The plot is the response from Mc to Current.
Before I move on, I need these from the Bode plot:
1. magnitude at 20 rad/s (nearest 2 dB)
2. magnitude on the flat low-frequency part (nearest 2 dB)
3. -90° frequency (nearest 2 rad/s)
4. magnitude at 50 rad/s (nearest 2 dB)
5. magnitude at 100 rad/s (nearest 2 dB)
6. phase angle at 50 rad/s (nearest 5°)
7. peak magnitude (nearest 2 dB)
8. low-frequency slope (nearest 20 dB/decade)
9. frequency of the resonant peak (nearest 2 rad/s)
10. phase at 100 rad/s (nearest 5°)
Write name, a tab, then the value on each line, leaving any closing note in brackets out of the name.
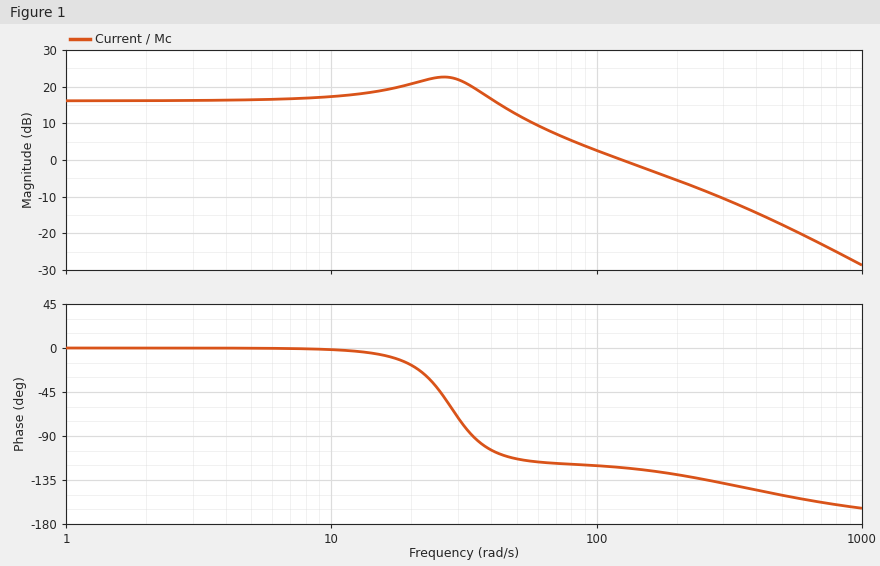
magnitude at 20 rad/s	20 dB
magnitude on the flat low-frequency part	16 dB
-90° frequency	34 rad/s
magnitude at 50 rad/s	12 dB
magnitude at 100 rad/s	2 dB
phase angle at 50 rad/s	-115°
peak magnitude	22 dB
low-frequency slope	0 dB/decade
frequency of the resonant peak	26 rad/s
phase at 100 rad/s	-120°
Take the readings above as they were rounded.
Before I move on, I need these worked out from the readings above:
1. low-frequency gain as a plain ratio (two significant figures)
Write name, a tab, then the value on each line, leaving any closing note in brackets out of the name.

low-frequency gain as a plain ratio	6.3
